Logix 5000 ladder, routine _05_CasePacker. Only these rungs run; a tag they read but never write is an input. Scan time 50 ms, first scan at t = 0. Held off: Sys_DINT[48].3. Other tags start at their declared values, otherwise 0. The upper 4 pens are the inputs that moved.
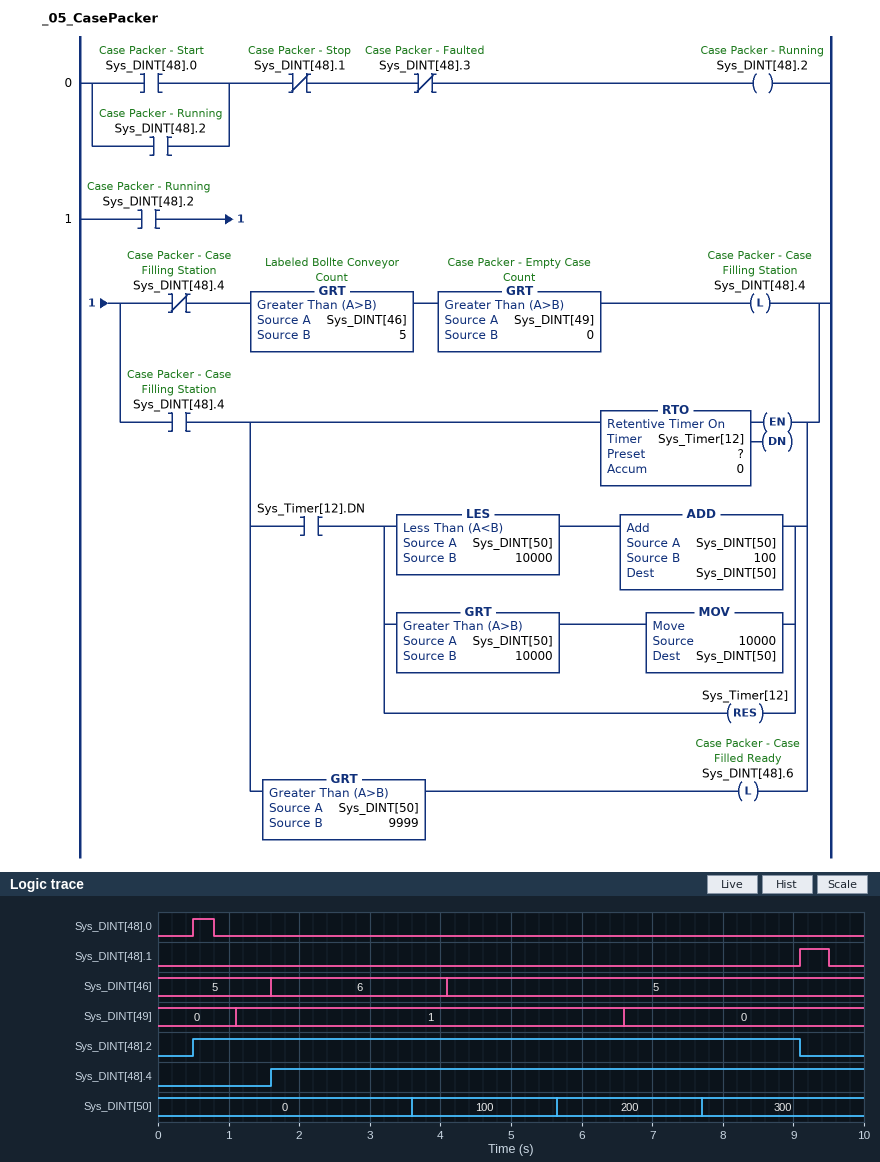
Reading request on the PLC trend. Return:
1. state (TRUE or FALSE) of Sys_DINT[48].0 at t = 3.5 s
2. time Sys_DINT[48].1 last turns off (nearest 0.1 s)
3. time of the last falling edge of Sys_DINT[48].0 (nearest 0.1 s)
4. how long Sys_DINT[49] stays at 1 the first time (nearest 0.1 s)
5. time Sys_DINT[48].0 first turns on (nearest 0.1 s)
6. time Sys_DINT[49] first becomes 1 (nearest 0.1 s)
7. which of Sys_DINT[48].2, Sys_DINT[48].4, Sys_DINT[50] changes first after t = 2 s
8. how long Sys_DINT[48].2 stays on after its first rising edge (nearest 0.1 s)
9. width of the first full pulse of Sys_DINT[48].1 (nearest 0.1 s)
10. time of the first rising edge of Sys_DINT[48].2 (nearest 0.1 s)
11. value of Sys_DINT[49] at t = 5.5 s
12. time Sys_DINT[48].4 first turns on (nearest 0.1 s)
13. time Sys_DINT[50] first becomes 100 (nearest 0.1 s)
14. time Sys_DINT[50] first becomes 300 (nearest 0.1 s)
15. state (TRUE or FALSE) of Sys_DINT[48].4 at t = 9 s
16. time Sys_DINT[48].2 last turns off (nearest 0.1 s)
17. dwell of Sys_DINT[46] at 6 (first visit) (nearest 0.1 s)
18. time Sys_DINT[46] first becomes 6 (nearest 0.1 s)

FALSE
9.5 s
0.8 s
5.5 s
0.5 s
1.1 s
Sys_DINT[50]
8.6 s
0.4 s
0.5 s
1
1.6 s
3.6 s
7.7 s
TRUE
9.1 s
2.5 s
1.6 s
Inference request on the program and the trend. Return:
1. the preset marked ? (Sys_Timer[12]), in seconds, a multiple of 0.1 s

2.0 s
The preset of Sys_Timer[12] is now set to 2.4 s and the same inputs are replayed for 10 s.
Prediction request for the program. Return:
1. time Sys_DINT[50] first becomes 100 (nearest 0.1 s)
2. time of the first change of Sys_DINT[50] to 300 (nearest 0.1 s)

4.0 s
8.9 s
